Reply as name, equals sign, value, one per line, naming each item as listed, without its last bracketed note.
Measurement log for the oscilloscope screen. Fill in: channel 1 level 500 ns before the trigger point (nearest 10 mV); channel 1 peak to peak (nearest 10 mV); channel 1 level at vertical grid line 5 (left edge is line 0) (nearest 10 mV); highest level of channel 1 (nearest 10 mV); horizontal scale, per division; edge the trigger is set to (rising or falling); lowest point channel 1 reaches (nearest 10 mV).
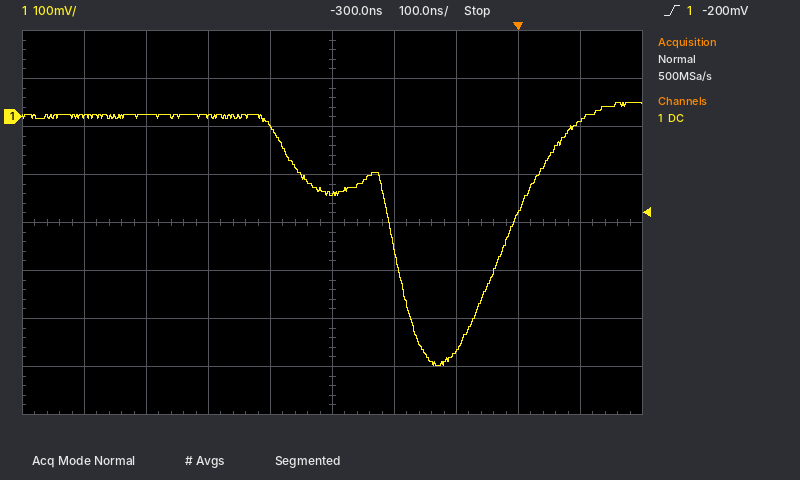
channel 1 level 500 ns before the trigger point = 0 mV
channel 1 peak to peak = 550 mV
channel 1 level at vertical grid line 5 (left edge is line 0) = -160 mV
highest level of channel 1 = 30 mV
horizontal scale, per division = 100 ns
edge the trigger is set to = rising
lowest point channel 1 reaches = -520 mV
